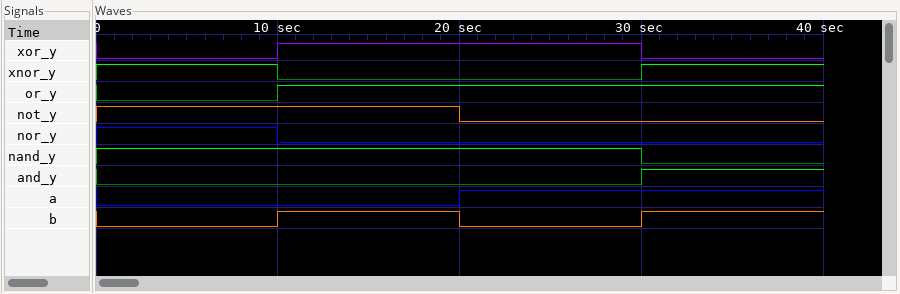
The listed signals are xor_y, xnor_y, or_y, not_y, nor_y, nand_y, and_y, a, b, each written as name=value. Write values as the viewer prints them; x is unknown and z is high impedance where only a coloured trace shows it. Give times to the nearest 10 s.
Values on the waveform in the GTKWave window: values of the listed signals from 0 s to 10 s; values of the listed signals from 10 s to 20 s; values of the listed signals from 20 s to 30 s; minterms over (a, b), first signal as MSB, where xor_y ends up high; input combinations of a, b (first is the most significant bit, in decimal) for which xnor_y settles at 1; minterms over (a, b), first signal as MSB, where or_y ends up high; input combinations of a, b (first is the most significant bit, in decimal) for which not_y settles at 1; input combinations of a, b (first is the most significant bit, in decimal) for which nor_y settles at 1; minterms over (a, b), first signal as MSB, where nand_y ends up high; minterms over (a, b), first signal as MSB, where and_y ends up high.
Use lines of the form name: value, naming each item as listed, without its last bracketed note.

values of the listed signals from 0 s to 10 s: xor_y=0, xnor_y=1, or_y=0, not_y=1, nor_y=1, nand_y=1, and_y=0, a=0, b=0
values of the listed signals from 10 s to 20 s: xor_y=1, xnor_y=0, or_y=1, not_y=1, nor_y=0, nand_y=1, and_y=0, a=0, b=1
values of the listed signals from 20 s to 30 s: xor_y=1, xnor_y=0, or_y=1, not_y=0, nor_y=0, nand_y=1, and_y=0, a=1, b=0
minterms over (a, b), first signal as MSB, where xor_y ends up high: 1, 2
input combinations of a, b (first is the most significant bit, in decimal) for which xnor_y settles at 1: 0, 3
minterms over (a, b), first signal as MSB, where or_y ends up high: 1, 2, 3
input combinations of a, b (first is the most significant bit, in decimal) for which not_y settles at 1: 0, 1
input combinations of a, b (first is the most significant bit, in decimal) for which nor_y settles at 1: 0
minterms over (a, b), first signal as MSB, where nand_y ends up high: 0, 1, 2
minterms over (a, b), first signal as MSB, where and_y ends up high: 3
